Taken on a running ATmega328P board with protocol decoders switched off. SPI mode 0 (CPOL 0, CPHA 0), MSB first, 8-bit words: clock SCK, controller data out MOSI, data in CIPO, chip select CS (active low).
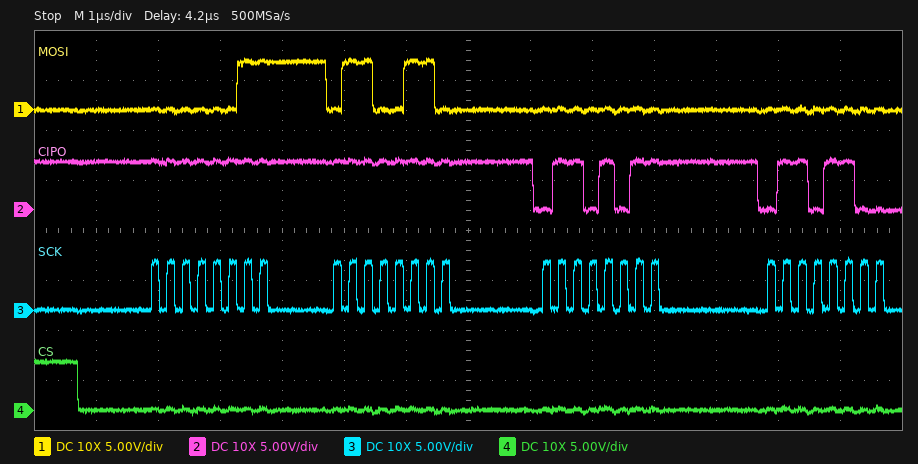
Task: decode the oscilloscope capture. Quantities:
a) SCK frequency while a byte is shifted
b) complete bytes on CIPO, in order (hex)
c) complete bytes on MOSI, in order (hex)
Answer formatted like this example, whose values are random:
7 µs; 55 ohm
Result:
4 MHz; FF FF 6B 6C; 03 66 00 00
